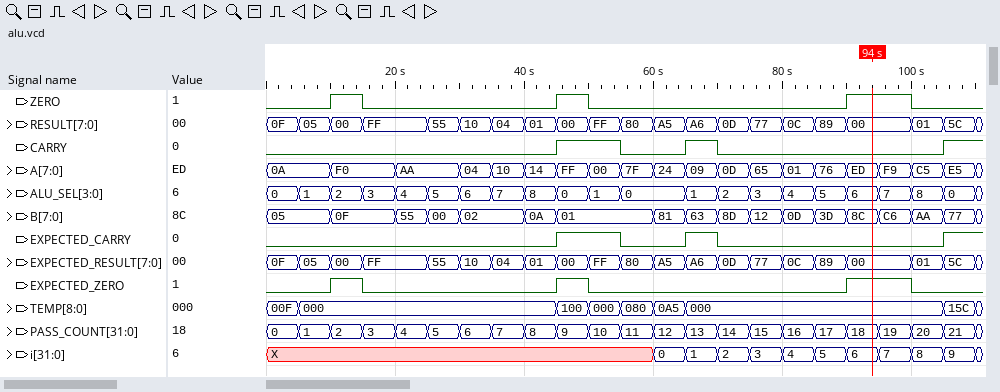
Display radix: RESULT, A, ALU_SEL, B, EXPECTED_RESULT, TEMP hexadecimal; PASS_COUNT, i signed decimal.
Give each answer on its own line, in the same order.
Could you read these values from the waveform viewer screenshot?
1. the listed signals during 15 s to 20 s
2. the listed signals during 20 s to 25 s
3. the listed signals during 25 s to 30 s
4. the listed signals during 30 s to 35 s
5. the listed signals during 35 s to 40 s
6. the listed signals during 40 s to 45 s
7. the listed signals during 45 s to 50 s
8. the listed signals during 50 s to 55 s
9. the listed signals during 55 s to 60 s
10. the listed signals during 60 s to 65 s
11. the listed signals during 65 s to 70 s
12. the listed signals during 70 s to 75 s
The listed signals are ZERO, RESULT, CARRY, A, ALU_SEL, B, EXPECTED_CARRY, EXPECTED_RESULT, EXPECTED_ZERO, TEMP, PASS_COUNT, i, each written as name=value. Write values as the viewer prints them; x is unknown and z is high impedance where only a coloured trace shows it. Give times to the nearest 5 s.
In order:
ZERO=0, RESULT=FF, CARRY=0, A=F0, ALU_SEL=3, B=0F, EXPECTED_CARRY=0, EXPECTED_RESULT=FF, EXPECTED_ZERO=0, TEMP=000, PASS_COUNT=3, i=X
ZERO=0, RESULT=FF, CARRY=0, A=AA, ALU_SEL=4, B=55, EXPECTED_CARRY=0, EXPECTED_RESULT=FF, EXPECTED_ZERO=0, TEMP=000, PASS_COUNT=4, i=X
ZERO=0, RESULT=55, CARRY=0, A=AA, ALU_SEL=5, B=00, EXPECTED_CARRY=0, EXPECTED_RESULT=55, EXPECTED_ZERO=0, TEMP=000, PASS_COUNT=5, i=X
ZERO=0, RESULT=10, CARRY=0, A=04, ALU_SEL=6, B=02, EXPECTED_CARRY=0, EXPECTED_RESULT=10, EXPECTED_ZERO=0, TEMP=000, PASS_COUNT=6, i=X
ZERO=0, RESULT=04, CARRY=0, A=10, ALU_SEL=7, B=02, EXPECTED_CARRY=0, EXPECTED_RESULT=04, EXPECTED_ZERO=0, TEMP=000, PASS_COUNT=7, i=X
ZERO=0, RESULT=01, CARRY=0, A=14, ALU_SEL=8, B=0A, EXPECTED_CARRY=0, EXPECTED_RESULT=01, EXPECTED_ZERO=0, TEMP=000, PASS_COUNT=8, i=X
ZERO=1, RESULT=00, CARRY=1, A=FF, ALU_SEL=0, B=01, EXPECTED_CARRY=1, EXPECTED_RESULT=00, EXPECTED_ZERO=1, TEMP=100, PASS_COUNT=9, i=X
ZERO=0, RESULT=FF, CARRY=1, A=00, ALU_SEL=1, B=01, EXPECTED_CARRY=1, EXPECTED_RESULT=FF, EXPECTED_ZERO=0, TEMP=000, PASS_COUNT=10, i=X
ZERO=0, RESULT=80, CARRY=0, A=7F, ALU_SEL=0, B=01, EXPECTED_CARRY=0, EXPECTED_RESULT=80, EXPECTED_ZERO=0, TEMP=080, PASS_COUNT=11, i=X
ZERO=0, RESULT=A5, CARRY=0, A=24, ALU_SEL=0, B=81, EXPECTED_CARRY=0, EXPECTED_RESULT=A5, EXPECTED_ZERO=0, TEMP=0A5, PASS_COUNT=12, i=0
ZERO=0, RESULT=A6, CARRY=1, A=09, ALU_SEL=1, B=63, EXPECTED_CARRY=1, EXPECTED_RESULT=A6, EXPECTED_ZERO=0, TEMP=000, PASS_COUNT=13, i=1
ZERO=0, RESULT=0D, CARRY=0, A=0D, ALU_SEL=2, B=8D, EXPECTED_CARRY=0, EXPECTED_RESULT=0D, EXPECTED_ZERO=0, TEMP=000, PASS_COUNT=14, i=2
